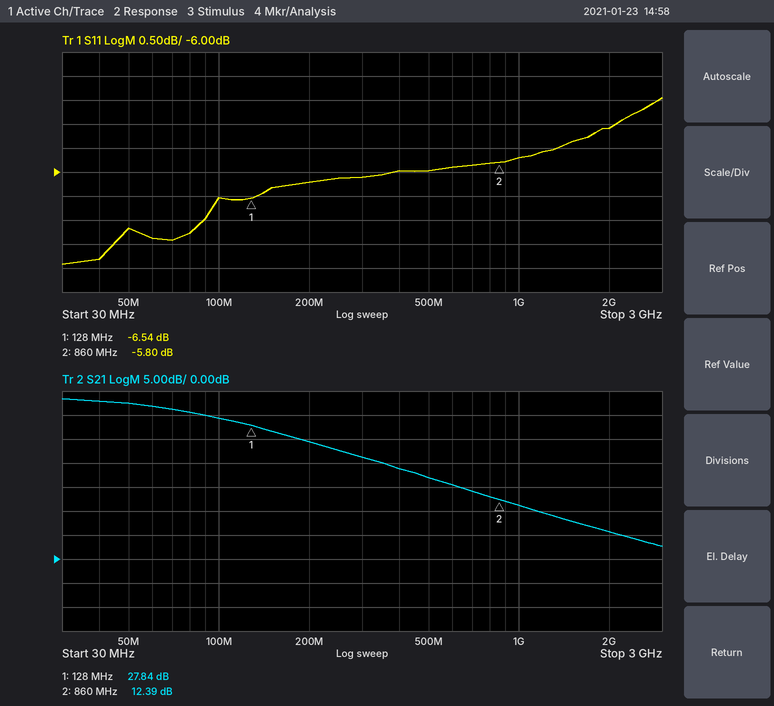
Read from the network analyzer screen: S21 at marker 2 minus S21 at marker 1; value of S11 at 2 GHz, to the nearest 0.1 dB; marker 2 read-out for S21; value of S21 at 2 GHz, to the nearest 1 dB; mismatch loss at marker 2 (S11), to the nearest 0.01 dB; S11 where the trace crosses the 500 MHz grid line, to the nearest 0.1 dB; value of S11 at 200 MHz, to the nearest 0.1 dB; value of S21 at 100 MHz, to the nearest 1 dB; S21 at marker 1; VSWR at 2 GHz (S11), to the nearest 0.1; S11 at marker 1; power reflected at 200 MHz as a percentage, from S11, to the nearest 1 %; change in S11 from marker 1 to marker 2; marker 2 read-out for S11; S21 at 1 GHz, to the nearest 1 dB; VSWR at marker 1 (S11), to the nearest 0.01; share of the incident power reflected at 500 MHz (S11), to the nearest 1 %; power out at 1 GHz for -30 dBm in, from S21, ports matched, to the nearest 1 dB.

-15.45 dB
-5.1 dB
12.39 dB
6 dB
1.33 dB
-6.0 dB
-6.2 dB
29 dB
27.84 dB
3.5
-6.54 dB
24 %
0.74 dB
-5.80 dB
11 dB
2.78
25 %
-19 dBm
